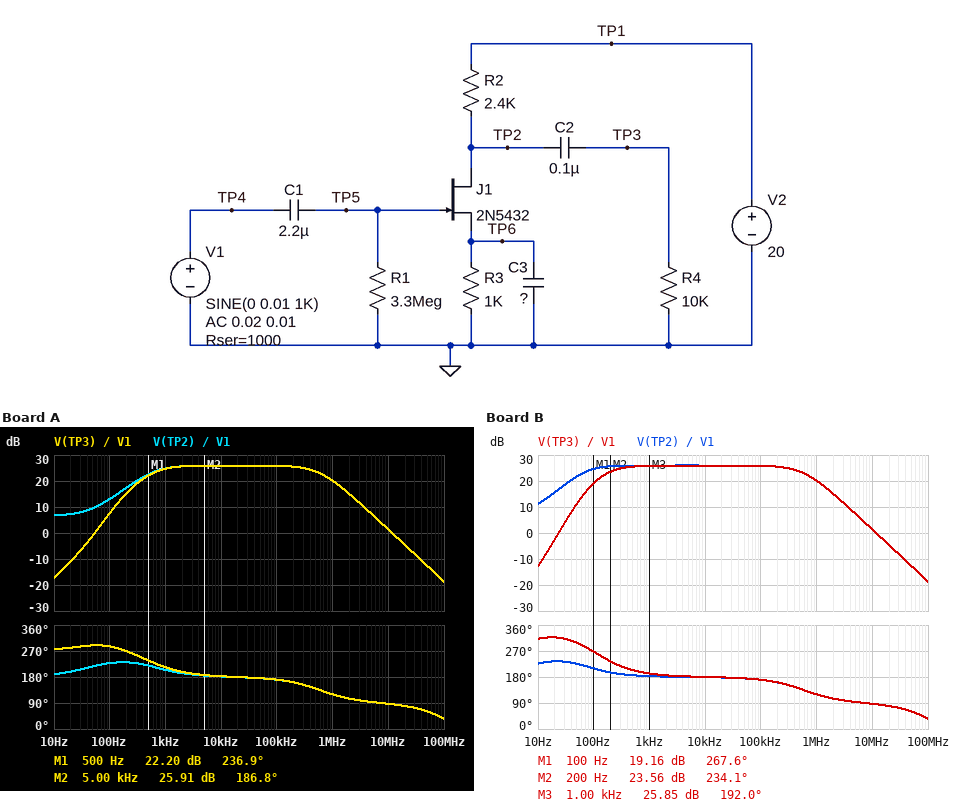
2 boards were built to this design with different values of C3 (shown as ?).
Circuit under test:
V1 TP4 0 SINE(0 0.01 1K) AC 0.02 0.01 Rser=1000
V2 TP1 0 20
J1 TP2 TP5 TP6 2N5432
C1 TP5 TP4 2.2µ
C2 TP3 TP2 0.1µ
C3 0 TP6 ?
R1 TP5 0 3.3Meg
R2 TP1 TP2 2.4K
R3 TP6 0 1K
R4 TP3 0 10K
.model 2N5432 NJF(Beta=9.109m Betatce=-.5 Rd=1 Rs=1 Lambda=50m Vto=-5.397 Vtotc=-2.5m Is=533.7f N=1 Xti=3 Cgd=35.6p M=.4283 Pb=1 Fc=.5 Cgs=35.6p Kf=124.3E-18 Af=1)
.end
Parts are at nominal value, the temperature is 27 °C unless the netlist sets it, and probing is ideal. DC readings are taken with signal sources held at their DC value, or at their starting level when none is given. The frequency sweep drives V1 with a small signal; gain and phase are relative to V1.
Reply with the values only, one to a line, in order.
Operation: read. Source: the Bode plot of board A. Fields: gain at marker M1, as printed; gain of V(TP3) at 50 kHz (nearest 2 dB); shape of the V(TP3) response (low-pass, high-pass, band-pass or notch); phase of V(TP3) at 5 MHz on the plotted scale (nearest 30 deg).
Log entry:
22.20 dB
26 dB
band-pass
90 deg
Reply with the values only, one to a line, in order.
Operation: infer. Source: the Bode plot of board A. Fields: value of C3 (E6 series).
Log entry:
3.3 µF
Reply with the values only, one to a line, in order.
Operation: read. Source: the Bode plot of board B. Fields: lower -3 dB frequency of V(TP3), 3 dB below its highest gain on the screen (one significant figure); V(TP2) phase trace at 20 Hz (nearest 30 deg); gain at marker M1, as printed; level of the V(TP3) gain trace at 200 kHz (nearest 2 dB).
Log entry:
200 Hz
240 deg
19.16 dB
26 dB
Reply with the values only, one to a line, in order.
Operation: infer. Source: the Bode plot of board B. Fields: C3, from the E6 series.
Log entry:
22 µF
